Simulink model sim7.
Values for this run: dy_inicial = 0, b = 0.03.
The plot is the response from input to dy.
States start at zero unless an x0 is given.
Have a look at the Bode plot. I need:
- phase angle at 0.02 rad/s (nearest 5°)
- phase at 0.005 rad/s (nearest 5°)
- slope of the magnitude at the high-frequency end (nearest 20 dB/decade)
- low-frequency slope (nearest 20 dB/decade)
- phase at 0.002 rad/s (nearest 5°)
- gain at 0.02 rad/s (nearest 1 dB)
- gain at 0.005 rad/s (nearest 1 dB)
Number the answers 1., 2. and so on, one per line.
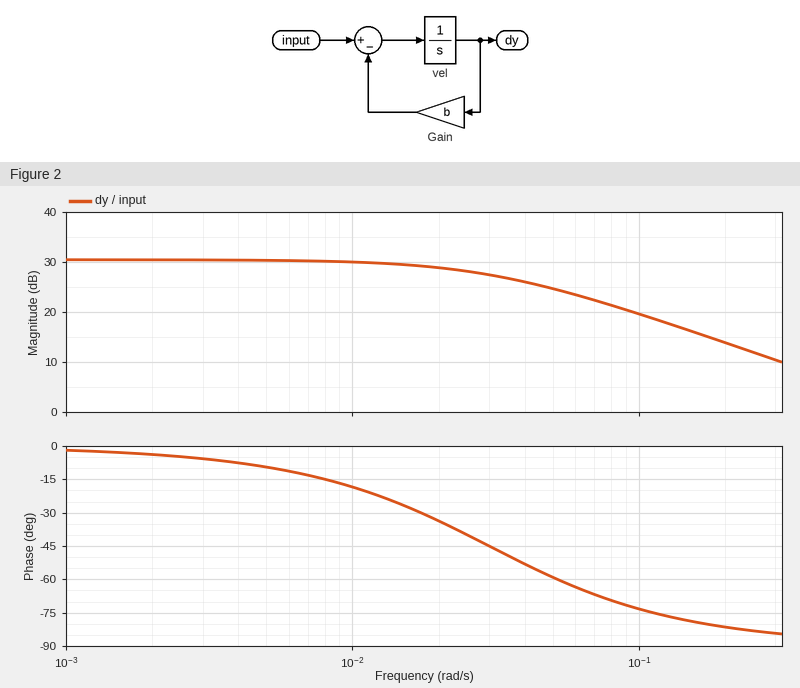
1. -35°
2. -10°
3. -20 dB/decade
4. 0 dB/decade
5. -5°
6. 29 dB
7. 30 dB
